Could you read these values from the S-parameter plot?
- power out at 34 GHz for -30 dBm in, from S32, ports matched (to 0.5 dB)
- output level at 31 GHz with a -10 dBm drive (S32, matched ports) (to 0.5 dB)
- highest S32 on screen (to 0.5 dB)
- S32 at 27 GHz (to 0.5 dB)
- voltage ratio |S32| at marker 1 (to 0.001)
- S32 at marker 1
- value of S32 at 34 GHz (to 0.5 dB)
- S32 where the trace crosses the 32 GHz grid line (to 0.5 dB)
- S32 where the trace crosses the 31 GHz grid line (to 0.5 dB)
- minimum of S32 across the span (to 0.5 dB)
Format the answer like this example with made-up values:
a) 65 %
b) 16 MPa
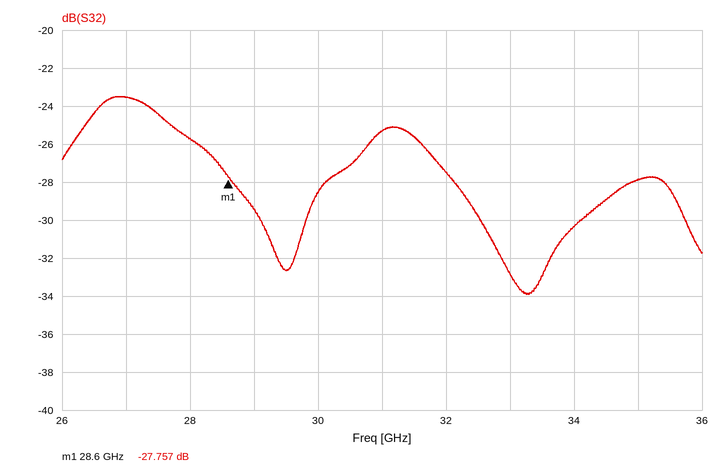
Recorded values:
a) -60.5 dBm
b) -35.5 dBm
c) -23.5 dB
d) -23.5 dB
e) 0.041
f) -27.757 dB
g) -30.5 dB
h) -27.5 dB
i) -25.5 dB
j) -34.0 dB
